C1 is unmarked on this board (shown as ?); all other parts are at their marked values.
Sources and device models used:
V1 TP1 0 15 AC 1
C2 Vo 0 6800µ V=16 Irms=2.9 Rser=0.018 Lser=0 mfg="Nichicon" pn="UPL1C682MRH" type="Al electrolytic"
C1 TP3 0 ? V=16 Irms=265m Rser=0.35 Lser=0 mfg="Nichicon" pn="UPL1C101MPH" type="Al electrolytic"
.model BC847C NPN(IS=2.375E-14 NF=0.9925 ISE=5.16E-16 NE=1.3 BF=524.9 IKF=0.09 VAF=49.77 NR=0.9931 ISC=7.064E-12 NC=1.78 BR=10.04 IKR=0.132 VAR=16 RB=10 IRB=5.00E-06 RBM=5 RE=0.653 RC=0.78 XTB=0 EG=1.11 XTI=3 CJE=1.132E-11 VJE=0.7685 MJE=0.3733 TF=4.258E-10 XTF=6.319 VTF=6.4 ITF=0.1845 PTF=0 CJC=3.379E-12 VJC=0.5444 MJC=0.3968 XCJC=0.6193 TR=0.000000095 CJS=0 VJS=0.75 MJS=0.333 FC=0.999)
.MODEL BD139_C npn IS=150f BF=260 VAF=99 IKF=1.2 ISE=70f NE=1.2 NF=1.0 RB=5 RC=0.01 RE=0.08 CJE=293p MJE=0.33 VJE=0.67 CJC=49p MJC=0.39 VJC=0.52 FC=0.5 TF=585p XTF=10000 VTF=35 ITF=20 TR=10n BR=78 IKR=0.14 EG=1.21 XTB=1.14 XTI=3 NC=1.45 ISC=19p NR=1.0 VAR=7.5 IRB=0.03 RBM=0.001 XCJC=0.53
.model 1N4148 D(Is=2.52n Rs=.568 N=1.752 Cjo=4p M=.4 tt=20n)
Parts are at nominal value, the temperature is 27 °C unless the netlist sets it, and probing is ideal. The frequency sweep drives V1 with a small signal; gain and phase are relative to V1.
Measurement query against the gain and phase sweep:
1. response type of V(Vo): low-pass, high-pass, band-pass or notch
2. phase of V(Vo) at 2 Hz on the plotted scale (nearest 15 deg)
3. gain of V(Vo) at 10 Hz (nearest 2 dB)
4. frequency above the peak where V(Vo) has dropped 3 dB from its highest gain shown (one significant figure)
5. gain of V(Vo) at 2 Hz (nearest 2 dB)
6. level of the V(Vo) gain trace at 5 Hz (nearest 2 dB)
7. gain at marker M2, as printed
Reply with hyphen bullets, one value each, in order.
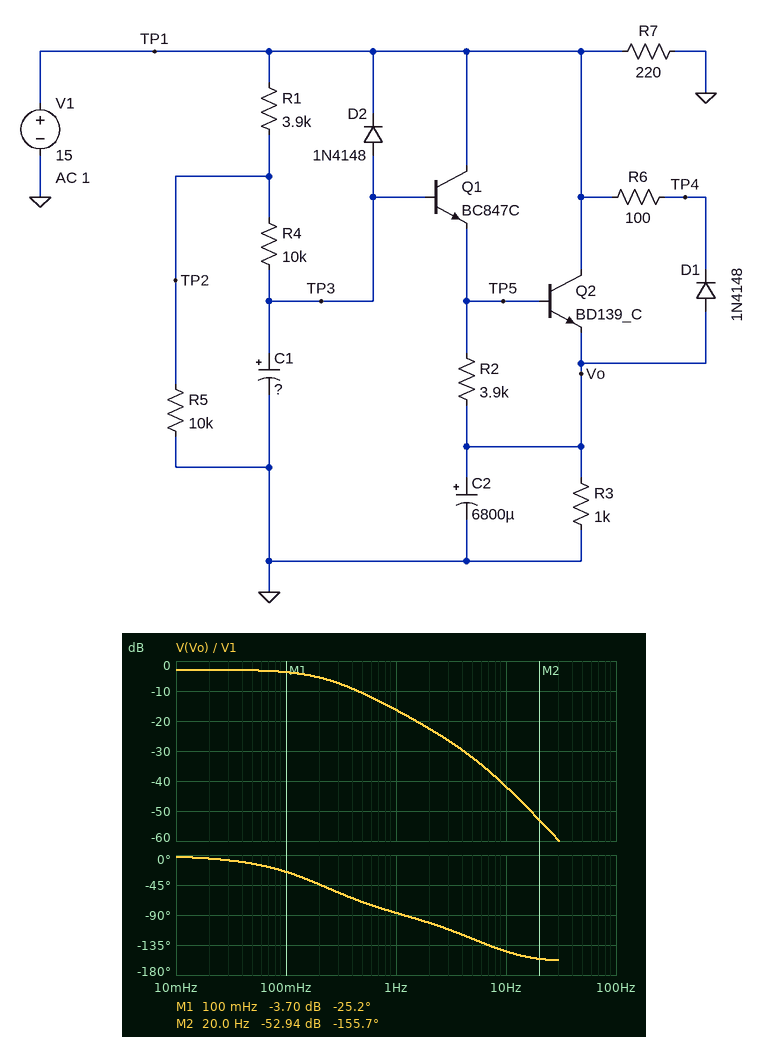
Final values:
- low-pass
- -105 deg
- -42 dB
- 200 mHz
- -22 dB
- -32 dB
- -52.94 dB
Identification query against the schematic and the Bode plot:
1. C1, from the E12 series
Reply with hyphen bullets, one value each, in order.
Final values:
- 56 µF
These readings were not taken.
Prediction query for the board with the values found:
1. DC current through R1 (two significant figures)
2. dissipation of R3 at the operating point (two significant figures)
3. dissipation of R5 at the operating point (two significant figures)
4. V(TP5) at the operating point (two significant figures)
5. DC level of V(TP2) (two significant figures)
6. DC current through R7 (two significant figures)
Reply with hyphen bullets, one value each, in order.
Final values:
- 1.1 mA
- 91 mW
- 12 mW
- 10 V
- 11 V
- 68 mA
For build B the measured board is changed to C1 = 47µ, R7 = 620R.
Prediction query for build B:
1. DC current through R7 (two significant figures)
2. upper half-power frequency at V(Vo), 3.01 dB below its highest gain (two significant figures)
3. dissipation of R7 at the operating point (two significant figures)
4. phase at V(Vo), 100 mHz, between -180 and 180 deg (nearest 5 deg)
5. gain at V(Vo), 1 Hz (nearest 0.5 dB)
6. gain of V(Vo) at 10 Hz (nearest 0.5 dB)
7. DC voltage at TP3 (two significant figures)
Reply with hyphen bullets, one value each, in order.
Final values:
- 24 mA
- 260 mHz
- 360 mW
- -20 deg
- -15.0 dB
- -40.5 dB
- 11 V
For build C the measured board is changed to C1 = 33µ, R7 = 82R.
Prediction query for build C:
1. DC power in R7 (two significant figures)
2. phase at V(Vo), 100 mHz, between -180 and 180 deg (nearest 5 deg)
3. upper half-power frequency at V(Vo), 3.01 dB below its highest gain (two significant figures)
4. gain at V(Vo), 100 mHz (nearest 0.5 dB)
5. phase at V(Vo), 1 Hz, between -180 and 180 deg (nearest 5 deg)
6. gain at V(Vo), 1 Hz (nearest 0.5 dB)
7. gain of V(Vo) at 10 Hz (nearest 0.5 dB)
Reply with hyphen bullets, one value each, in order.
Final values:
- 2.7 W
- -15 deg
- 370 mHz
- -3.0 dB
- -80 deg
- -12.0 dB
- -37.5 dB
